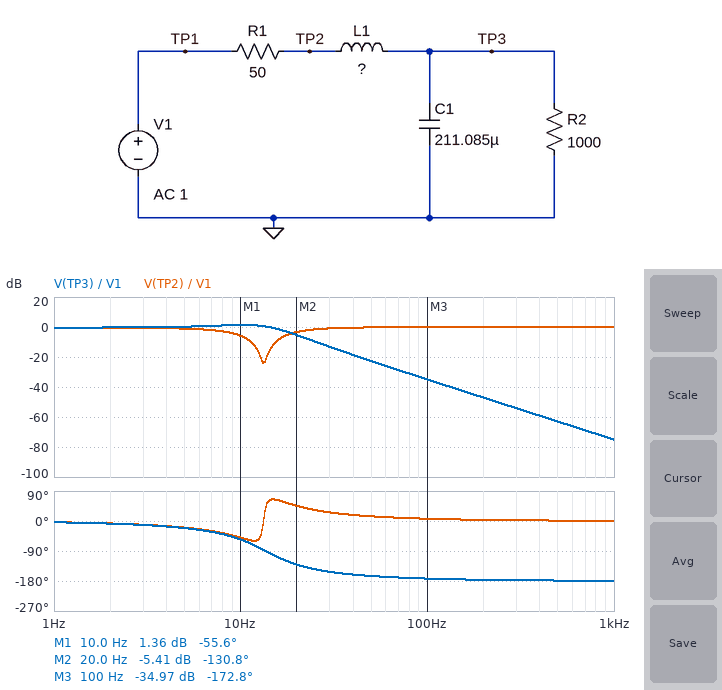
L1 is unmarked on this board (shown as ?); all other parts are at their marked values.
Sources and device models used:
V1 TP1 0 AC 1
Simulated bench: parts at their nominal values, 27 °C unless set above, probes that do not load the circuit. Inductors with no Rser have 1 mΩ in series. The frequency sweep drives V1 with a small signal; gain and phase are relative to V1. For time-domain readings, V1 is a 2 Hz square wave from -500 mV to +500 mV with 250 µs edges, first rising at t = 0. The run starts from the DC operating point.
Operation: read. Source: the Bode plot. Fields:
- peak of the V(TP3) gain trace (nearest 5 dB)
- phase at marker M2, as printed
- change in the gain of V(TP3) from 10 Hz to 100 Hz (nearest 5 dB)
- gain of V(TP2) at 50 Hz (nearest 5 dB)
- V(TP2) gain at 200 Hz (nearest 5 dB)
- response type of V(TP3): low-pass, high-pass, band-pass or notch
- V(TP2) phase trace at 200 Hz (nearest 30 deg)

0 dB
-130.8 deg
-35 dB
0 dB
0 dB
low-pass
0 deg
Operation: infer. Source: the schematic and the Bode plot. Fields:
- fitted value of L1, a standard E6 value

680 mH
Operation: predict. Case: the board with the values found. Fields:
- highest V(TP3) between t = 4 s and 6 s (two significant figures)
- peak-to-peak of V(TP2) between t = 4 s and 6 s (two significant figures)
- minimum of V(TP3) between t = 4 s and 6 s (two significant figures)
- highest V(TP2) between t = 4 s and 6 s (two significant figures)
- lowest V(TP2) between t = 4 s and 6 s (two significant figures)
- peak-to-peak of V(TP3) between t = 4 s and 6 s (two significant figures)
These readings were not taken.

670 mV
1.1 V
-670 mV
570 mV
-570 mV
1.3 V
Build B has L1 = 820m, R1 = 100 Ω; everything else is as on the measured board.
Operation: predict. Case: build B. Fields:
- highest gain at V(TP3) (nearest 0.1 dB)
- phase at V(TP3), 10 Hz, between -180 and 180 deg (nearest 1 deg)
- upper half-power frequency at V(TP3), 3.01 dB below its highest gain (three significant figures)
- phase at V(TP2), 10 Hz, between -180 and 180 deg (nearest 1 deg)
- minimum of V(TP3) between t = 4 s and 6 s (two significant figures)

-0.8 dB
-73 deg
11.1 Hz
-64 deg
-470 mV
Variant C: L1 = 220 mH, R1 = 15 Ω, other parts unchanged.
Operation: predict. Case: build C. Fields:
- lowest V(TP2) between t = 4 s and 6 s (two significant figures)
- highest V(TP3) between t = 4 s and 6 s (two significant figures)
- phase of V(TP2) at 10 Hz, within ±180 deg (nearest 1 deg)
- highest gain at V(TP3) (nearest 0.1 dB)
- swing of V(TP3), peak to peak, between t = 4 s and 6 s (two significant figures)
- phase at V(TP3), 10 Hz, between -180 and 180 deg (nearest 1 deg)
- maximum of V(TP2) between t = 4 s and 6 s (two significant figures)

-640 mV
940 mV
-13 deg
6.3 dB
1.9 V
-14 deg
640 mV
